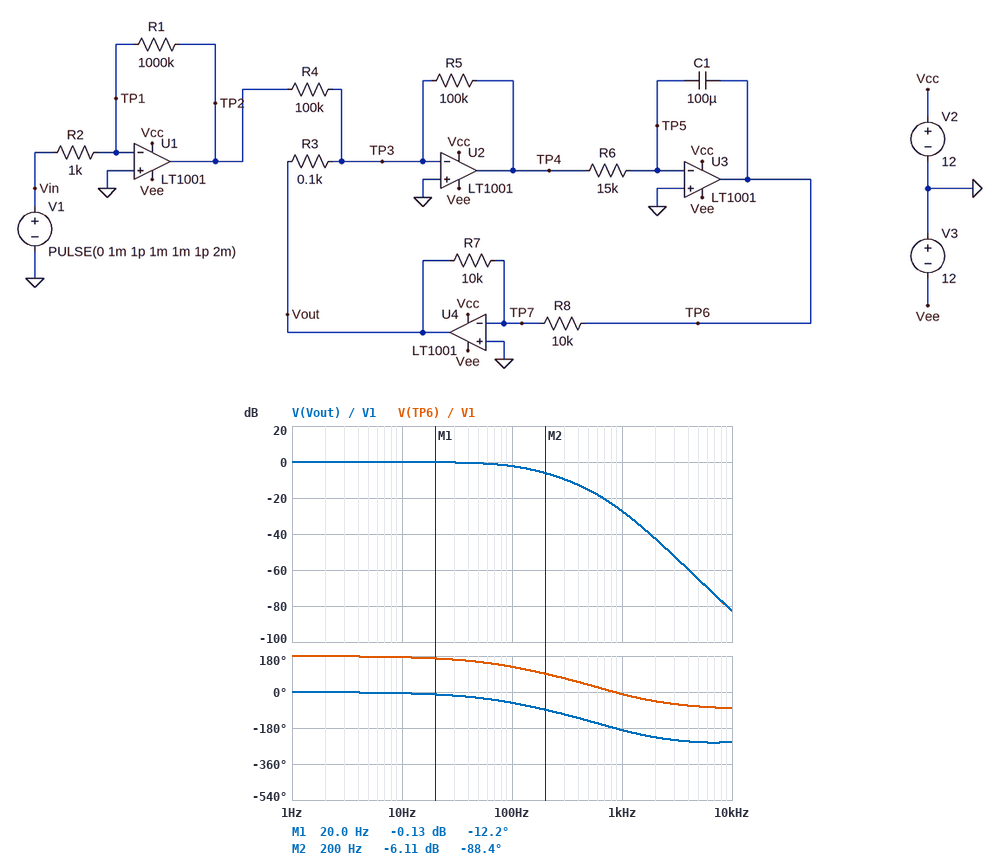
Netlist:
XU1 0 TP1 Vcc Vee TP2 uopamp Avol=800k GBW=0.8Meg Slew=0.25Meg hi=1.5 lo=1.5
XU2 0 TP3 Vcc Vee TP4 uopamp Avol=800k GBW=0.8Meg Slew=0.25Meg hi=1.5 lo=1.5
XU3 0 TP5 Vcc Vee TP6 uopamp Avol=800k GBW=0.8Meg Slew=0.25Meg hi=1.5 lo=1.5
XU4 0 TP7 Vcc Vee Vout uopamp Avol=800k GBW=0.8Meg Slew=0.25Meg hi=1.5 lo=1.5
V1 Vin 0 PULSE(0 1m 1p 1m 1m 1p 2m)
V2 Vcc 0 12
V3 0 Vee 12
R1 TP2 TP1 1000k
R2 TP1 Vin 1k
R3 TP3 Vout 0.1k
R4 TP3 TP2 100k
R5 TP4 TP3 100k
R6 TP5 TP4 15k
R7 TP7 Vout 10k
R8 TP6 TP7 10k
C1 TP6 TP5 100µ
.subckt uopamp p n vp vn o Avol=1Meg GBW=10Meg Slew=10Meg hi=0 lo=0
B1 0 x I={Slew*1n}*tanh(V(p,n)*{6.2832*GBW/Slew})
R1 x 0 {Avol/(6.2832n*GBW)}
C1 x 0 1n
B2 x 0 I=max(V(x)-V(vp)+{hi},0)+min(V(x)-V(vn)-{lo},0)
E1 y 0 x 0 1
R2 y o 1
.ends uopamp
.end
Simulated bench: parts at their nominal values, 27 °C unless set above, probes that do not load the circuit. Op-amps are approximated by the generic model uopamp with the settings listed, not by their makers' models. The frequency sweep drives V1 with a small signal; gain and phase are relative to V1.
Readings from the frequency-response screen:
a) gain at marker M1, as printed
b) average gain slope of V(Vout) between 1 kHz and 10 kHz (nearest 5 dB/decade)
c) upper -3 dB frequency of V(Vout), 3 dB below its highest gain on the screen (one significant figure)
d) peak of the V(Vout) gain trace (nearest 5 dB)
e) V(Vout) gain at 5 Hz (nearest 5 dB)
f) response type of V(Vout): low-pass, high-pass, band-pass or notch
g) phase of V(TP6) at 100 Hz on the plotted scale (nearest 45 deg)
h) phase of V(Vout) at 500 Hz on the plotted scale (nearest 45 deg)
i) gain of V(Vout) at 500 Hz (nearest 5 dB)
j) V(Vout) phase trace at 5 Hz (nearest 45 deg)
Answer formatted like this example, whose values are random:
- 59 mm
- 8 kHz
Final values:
- -0.13 dB
- -55 dB/decade
- 100 Hz
- 0 dB
- 0 dB
- low-pass
- 135 deg
- -135 deg
- -15 dB
- 0 deg
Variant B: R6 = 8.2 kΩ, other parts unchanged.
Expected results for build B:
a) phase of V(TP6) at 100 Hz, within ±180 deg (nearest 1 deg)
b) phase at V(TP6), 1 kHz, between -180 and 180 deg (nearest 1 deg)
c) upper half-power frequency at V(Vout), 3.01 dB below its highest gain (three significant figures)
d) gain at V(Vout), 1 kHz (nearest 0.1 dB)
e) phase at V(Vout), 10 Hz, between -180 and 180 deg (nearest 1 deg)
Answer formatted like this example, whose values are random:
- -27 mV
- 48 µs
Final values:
- 144 deg
- -8 deg
- 231 Hz
- -21.6 dB
- -4 deg
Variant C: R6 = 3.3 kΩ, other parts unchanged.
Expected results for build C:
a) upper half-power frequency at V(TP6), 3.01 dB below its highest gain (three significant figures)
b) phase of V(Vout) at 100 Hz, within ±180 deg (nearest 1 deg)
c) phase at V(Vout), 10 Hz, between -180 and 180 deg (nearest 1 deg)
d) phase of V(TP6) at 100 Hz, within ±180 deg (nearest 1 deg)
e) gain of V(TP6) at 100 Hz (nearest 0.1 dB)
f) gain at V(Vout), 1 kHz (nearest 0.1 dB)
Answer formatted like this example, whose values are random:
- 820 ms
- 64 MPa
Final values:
- 553 Hz
- -19 deg
- -2 deg
- 161 deg
- 0 dB
- -12.4 dB
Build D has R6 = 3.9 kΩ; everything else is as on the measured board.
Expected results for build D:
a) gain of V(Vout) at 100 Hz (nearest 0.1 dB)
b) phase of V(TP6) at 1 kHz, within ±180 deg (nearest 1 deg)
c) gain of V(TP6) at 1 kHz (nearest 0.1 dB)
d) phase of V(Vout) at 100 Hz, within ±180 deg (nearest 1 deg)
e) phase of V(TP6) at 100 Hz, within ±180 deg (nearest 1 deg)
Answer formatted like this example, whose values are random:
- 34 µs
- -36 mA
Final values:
- -0.1 dB
- -2 deg
- -14.2 dB
- -21 deg
- 159 deg
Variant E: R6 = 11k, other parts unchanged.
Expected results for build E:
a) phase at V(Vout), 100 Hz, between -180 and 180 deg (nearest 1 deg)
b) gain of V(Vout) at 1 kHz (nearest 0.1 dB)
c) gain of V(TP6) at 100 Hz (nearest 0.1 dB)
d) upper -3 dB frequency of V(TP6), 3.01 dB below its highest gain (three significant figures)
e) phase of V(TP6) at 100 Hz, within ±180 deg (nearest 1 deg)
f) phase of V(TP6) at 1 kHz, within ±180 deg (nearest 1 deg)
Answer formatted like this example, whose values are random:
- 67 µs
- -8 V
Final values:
- -44 deg
- -24.4 dB
- -1.3 dB
- 168 Hz
- 136 deg
- -9 deg
